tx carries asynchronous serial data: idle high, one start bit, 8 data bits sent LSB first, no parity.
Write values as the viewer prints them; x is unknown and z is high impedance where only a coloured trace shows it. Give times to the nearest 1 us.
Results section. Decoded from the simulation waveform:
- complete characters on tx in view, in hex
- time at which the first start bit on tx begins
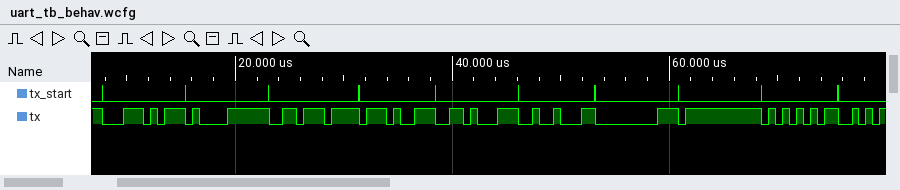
5C, E1, 76, 97, 16, 12, 00, FF, 55
8 us
